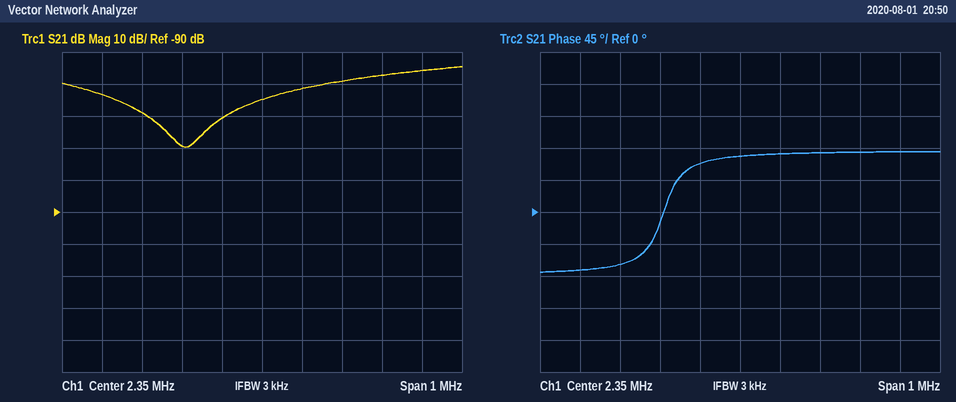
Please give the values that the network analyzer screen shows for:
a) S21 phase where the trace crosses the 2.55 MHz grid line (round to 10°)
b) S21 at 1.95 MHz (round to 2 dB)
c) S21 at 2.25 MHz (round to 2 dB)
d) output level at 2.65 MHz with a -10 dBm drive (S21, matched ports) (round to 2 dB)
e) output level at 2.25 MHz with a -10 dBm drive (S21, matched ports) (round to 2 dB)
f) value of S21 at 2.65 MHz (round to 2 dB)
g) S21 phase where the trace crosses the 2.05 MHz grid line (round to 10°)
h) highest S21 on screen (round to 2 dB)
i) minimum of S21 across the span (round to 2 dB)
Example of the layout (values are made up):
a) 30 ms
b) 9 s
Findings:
a) 80°
b) -54 dB
c) -60 dB
d) -58 dBm
e) -70 dBm
f) -48 dB
g) -70°
h) -44 dB
i) -70 dB
